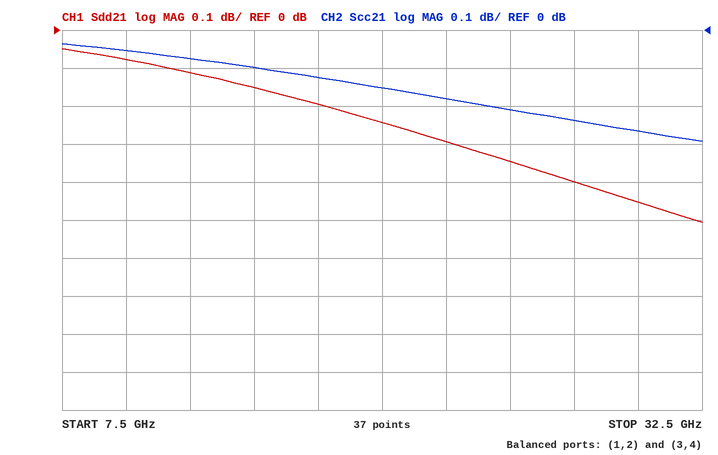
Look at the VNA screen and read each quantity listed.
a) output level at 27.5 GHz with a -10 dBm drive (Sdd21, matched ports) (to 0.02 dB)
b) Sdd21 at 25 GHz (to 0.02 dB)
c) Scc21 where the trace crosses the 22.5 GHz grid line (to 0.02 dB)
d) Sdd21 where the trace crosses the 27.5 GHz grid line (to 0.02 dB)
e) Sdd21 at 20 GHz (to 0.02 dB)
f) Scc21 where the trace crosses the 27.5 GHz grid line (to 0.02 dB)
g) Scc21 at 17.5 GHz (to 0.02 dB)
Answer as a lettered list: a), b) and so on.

a) -10.40 dBm
b) -0.34 dB
c) -0.18 dB
d) -0.40 dB
e) -0.24 dB
f) -0.24 dB
g) -0.12 dB
